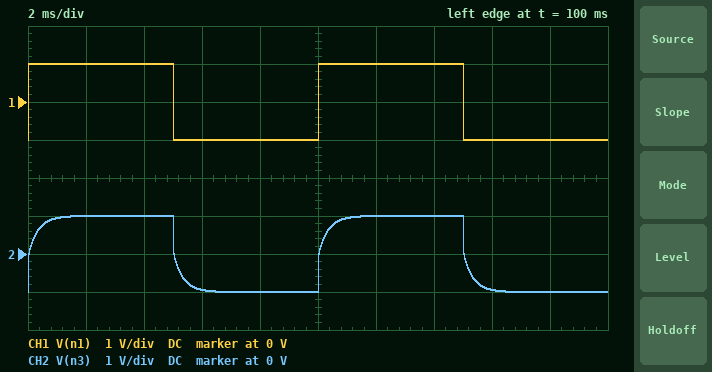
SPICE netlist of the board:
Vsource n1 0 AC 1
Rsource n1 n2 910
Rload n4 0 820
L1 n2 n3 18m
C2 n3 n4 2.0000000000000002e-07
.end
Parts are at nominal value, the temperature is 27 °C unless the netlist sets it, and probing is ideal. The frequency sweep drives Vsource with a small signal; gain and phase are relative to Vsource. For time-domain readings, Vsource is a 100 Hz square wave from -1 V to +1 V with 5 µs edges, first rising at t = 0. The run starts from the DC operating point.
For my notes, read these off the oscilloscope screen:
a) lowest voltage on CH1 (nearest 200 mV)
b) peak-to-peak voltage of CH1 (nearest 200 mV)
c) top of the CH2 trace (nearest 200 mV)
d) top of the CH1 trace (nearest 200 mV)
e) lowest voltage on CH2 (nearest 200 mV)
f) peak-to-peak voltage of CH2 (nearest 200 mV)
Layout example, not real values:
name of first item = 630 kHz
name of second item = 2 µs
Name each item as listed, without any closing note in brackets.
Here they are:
lowest voltage on CH1 = -1.0 V
peak-to-peak voltage of CH1 = 2.0 V
top of the CH2 trace = 1.0 V
top of the CH1 trace = 1.0 V
lowest voltage on CH2 = -1.0 V
peak-to-peak voltage of CH2 = 2.0 V
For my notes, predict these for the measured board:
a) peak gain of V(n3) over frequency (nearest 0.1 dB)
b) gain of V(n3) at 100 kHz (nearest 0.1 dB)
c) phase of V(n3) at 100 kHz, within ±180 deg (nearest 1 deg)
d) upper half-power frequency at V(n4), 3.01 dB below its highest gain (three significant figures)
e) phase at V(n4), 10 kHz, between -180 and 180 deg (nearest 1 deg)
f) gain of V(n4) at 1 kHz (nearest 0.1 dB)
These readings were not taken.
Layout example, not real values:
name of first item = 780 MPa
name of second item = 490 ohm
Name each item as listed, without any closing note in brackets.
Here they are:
peak gain of V(n3) over frequency = 0 dB
gain of V(n3) at 100 kHz = -22.9 dB
phase of V(n3) at 100 kHz, within ±180 deg = -82 deg
upper half-power frequency at V(n4), 3.01 dB below its highest gain = 15.7 kHz
phase at V(n4), 10 kHz, between -180 and 180 deg = -31 deg
gain of V(n4) at 1 kHz = -7.1 dB
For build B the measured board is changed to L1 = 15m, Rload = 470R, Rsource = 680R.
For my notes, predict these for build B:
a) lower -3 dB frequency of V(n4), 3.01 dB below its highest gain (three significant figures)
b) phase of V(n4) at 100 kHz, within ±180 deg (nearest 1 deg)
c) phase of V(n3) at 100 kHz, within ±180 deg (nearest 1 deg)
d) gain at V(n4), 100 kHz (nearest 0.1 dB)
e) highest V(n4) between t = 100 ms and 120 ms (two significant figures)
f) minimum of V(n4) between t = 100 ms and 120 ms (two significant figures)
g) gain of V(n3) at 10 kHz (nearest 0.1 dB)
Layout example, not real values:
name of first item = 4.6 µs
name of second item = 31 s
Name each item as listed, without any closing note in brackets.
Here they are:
lower -3 dB frequency of V(n4), 3.01 dB below its highest gain = 657 Hz
phase of V(n4) at 100 kHz, within ±180 deg = -83 deg
phase of V(n3) at 100 kHz, within ±180 deg = -84 deg
gain at V(n4), 100 kHz = -26.1 dB
highest V(n4) between t = 100 ms and 120 ms = 730 mV
minimum of V(n4) between t = 100 ms and 120 ms = -730 mV
gain of V(n3) at 10 kHz = -9.6 dB
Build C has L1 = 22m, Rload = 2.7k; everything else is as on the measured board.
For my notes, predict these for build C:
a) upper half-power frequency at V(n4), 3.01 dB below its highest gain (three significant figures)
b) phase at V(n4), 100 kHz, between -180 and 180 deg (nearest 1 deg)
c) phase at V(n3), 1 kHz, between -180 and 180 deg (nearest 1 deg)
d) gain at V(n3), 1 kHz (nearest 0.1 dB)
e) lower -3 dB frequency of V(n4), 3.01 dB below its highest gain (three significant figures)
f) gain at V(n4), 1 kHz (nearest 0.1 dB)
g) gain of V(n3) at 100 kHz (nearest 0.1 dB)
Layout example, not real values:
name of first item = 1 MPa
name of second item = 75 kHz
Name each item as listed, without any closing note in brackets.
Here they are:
upper half-power frequency at V(n4), 3.01 dB below its highest gain = 26.3 kHz
phase at V(n4), 100 kHz, between -180 and 180 deg = -75 deg
phase at V(n3), 1 kHz, between -180 and 180 deg = -6 deg
gain at V(n3), 1 kHz = -2.3 dB
lower -3 dB frequency of V(n4), 3.01 dB below its highest gain = 219 Hz
gain at V(n4), 1 kHz = -2.7 dB
gain of V(n3) at 100 kHz = -14.5 dB
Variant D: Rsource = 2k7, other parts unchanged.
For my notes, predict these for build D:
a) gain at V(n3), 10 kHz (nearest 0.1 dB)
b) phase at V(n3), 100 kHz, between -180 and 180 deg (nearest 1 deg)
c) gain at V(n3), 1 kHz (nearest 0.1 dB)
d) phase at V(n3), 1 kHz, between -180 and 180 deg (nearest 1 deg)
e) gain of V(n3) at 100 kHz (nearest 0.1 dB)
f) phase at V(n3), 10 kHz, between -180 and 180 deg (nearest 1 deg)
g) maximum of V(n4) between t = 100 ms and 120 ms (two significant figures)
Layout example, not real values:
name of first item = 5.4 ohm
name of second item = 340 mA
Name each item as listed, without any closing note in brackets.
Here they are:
gain at V(n3), 10 kHz = -13.0 dB
phase at V(n3), 100 kHz, between -180 and 180 deg = -73 deg
gain at V(n3), 1 kHz = -9.9 dB
phase at V(n3), 1 kHz, between -180 and 180 deg = -33 deg
gain of V(n3) at 100 kHz = -23.2 dB
phase at V(n3), 10 kHz, between -180 and 180 deg = -22 deg
maximum of V(n4) between t = 100 ms and 120 ms = 450 mV
